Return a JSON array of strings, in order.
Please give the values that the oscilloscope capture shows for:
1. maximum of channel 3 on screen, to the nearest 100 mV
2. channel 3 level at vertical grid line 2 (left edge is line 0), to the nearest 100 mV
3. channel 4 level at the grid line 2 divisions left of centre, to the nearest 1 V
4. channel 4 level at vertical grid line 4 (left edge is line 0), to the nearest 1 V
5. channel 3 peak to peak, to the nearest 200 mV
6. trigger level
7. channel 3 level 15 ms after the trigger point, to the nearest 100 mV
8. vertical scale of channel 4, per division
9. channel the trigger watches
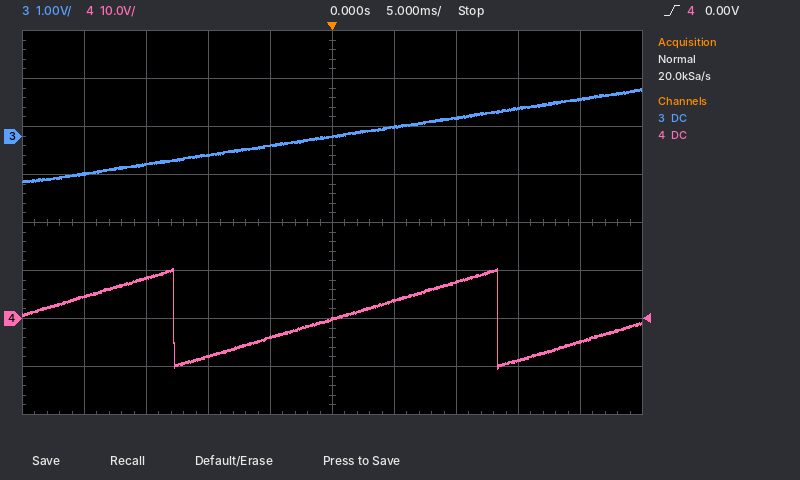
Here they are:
["1.0 V", "-600 mV", "-8 V", "-4 V", "2.0 V", "0.00 V", "600 mV", "10 V", "channel 4"]
